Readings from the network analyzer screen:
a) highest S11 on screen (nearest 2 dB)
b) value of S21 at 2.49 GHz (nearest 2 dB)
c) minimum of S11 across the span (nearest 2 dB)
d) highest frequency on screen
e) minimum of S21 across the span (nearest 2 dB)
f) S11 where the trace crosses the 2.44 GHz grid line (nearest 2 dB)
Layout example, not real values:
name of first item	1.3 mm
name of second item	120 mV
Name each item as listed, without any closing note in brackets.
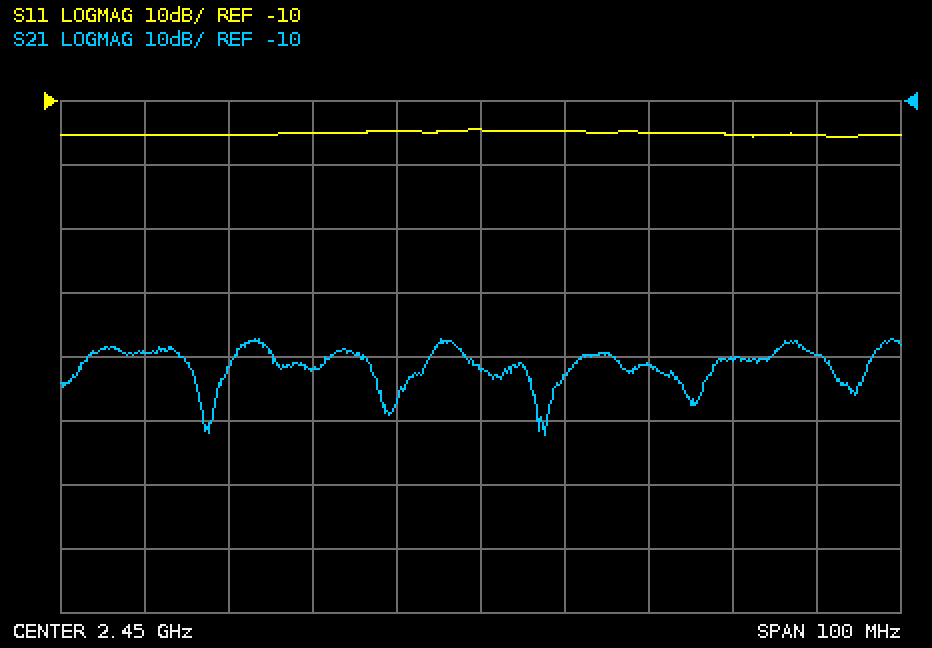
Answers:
highest S11 on screen	-14 dB
value of S21 at 2.49 GHz	-50 dB
minimum of S11 across the span	-16 dB
highest frequency on screen	2.5 GHz
minimum of S21 across the span	-62 dB
S11 where the trace crosses the 2.44 GHz grid line	-14 dB
